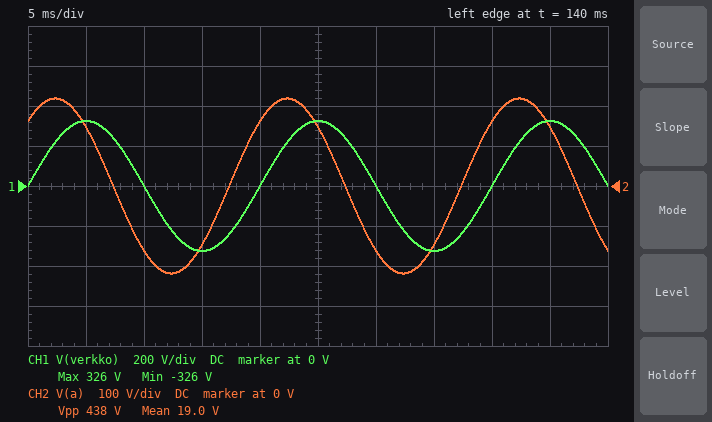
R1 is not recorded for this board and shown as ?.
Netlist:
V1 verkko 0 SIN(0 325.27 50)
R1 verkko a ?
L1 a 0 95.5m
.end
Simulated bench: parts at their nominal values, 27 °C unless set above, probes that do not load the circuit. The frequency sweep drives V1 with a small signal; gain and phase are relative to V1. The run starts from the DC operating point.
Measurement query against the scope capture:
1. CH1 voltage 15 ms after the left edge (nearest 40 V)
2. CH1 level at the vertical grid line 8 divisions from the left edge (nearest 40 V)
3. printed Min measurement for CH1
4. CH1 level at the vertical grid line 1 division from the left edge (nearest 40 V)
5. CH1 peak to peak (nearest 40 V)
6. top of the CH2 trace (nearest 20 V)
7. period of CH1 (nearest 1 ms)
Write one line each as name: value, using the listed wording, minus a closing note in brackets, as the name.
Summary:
CH1 voltage 15 ms after the left edge: -320 V
CH1 level at the vertical grid line 8 divisions from the left edge: 0 V
printed Min measurement for CH1: -326 V
CH1 level at the vertical grid line 1 division from the left edge: 320 V
CH1 peak to peak: 640 V
top of the CH2 trace: 220 V
period of CH1: 20 ms
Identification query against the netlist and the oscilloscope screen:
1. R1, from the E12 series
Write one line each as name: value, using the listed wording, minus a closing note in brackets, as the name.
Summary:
R1, from the E12 series: 33 Ω
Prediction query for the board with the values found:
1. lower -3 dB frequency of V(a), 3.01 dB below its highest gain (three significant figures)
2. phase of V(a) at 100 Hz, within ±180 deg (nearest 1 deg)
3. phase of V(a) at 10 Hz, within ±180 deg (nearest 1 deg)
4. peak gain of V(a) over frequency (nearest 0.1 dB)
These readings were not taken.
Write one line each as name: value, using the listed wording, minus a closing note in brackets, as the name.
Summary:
lower -3 dB frequency of V(a), 3.01 dB below its highest gain: 55.0 Hz
phase of V(a) at 100 Hz, within ±180 deg: 29 deg
phase of V(a) at 10 Hz, within ±180 deg: 80 deg
peak gain of V(a) over frequency: 0 dB
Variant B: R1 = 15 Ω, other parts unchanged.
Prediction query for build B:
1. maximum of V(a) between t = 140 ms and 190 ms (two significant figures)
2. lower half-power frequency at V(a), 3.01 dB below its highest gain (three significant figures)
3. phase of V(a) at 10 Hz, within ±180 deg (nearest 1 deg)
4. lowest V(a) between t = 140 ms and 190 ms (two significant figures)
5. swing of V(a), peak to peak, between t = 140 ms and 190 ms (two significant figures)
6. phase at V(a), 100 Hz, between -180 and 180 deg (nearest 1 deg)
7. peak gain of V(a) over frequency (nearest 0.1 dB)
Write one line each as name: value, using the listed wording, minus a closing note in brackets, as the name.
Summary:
maximum of V(a) between t = 140 ms and 190 ms: 290 V
lower half-power frequency at V(a), 3.01 dB below its highest gain: 25.0 Hz
phase of V(a) at 10 Hz, within ±180 deg: 68 deg
lowest V(a) between t = 140 ms and 190 ms: -290 V
swing of V(a), peak to peak, between t = 140 ms and 190 ms: 580 V
phase at V(a), 100 Hz, between -180 and 180 deg: 14 deg
peak gain of V(a) over frequency: 0 dB
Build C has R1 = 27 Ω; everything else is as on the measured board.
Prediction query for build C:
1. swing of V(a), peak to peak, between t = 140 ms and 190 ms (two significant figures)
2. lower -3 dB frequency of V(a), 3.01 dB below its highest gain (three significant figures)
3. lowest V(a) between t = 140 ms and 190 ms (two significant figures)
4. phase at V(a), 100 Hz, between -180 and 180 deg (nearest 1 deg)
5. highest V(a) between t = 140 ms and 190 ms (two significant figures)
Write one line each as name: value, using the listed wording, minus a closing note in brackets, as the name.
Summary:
swing of V(a), peak to peak, between t = 140 ms and 190 ms: 480 V
lower -3 dB frequency of V(a), 3.01 dB below its highest gain: 45.0 Hz
lowest V(a) between t = 140 ms and 190 ms: -240 V
phase at V(a), 100 Hz, between -180 and 180 deg: 24 deg
highest V(a) between t = 140 ms and 190 ms: 240 V
